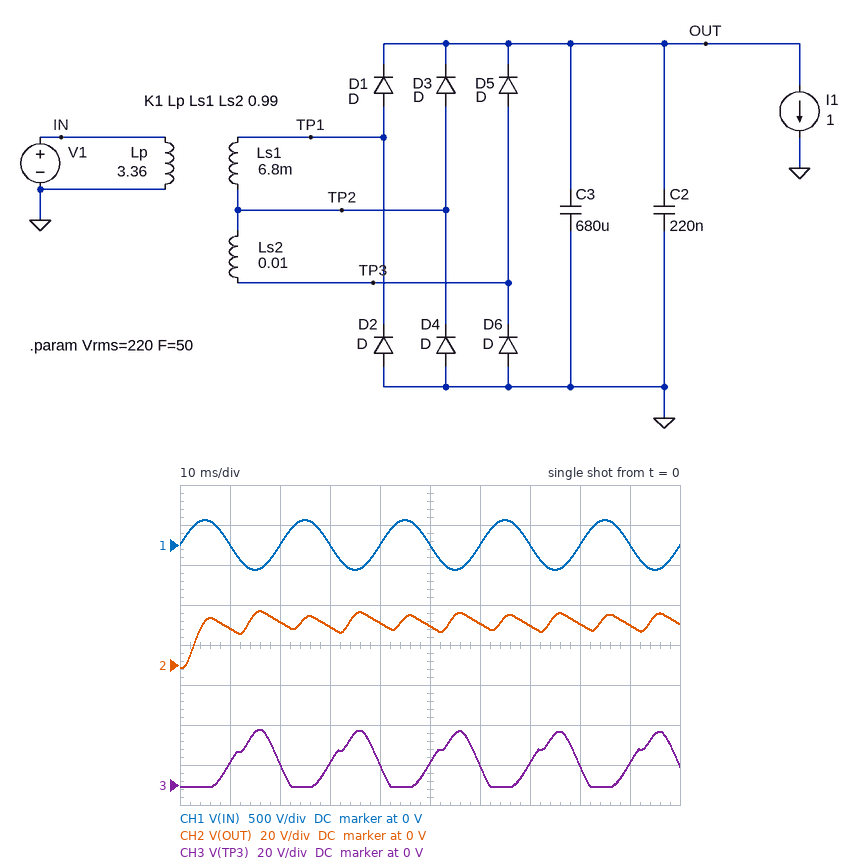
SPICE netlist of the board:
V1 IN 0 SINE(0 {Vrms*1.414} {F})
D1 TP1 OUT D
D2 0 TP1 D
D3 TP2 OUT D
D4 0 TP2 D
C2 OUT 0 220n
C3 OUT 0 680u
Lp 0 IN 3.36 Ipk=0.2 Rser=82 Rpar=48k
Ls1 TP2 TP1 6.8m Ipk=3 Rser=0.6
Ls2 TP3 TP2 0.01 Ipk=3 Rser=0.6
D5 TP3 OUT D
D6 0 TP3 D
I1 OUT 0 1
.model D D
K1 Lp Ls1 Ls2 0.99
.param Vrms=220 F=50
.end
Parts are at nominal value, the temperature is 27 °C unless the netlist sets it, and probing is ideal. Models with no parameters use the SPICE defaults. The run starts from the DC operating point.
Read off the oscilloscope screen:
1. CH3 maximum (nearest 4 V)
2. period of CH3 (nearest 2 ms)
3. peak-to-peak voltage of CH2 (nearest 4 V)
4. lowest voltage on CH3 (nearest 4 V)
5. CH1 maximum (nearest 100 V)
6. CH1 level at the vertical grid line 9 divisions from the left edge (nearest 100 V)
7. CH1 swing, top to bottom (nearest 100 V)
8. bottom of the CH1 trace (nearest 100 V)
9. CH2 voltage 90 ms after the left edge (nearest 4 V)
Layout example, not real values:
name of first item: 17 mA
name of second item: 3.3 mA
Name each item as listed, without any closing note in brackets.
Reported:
CH3 maximum: 28 V
period of CH3: 20 ms
peak-to-peak voltage of CH2: 28 V
lowest voltage on CH3: 0 V
CH1 maximum: 300 V
CH1 level at the vertical grid line 9 divisions from the left edge: 0 V
CH1 swing, top to bottom: 600 V
bottom of the CH1 trace: -300 V
CH2 voltage 90 ms after the left edge: 20 V
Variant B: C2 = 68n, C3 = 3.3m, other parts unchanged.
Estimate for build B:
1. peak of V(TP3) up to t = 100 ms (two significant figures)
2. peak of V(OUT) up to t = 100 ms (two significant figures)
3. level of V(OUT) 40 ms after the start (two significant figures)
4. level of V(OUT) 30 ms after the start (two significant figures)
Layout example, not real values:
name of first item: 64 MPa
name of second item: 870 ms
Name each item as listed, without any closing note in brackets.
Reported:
peak of V(TP3) up to t = 100 ms: 24 V
peak of V(OUT) up to t = 100 ms: 23 V
level of V(OUT) 40 ms after the start: 21 V
level of V(OUT) 30 ms after the start: 20 V
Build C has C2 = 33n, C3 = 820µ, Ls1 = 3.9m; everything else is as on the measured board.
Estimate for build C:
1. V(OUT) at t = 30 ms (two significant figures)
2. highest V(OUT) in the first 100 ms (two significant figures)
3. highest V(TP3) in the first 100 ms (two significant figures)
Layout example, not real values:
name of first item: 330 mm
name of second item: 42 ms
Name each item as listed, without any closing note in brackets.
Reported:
V(OUT) at t = 30 ms: 17 V
highest V(OUT) in the first 100 ms: 23 V
highest V(TP3) in the first 100 ms: 24 V
